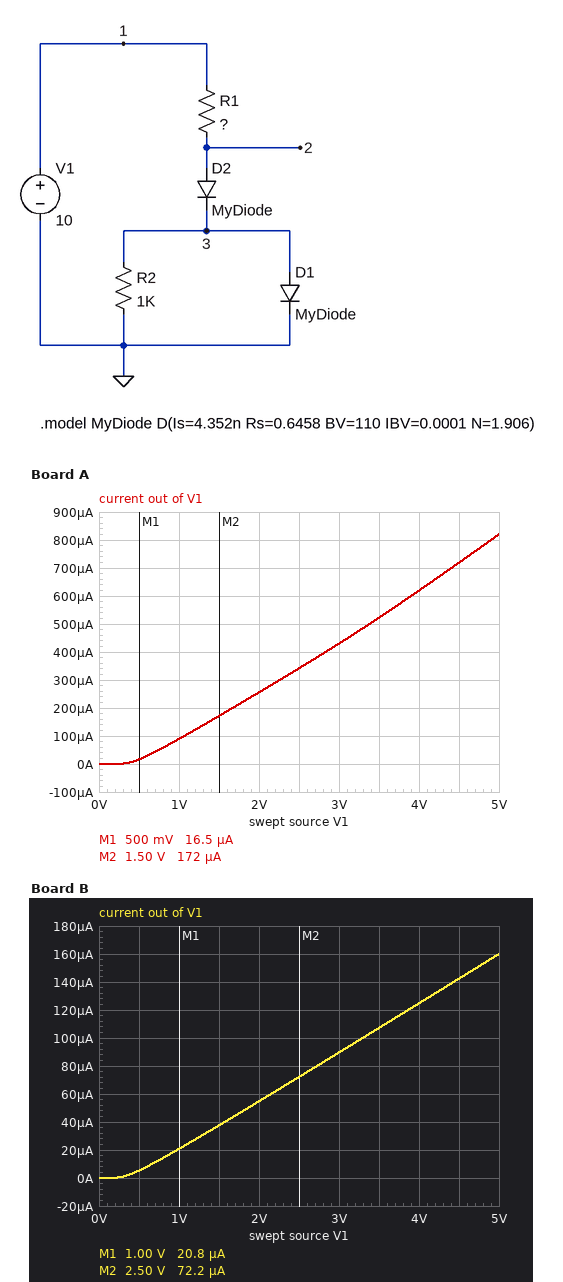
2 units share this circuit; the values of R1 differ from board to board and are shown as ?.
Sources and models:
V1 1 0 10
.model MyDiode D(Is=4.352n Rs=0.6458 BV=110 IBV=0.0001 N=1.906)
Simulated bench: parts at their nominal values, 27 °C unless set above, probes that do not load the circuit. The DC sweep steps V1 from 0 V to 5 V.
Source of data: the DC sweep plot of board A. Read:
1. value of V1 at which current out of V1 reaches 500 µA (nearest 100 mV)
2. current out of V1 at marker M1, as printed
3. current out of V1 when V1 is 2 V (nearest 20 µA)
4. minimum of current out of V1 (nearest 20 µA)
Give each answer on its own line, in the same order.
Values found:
3.4 V
16.5 µA
260 µA
0 A
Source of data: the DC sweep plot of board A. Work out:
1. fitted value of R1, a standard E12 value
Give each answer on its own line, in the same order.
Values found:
4.7 kΩ
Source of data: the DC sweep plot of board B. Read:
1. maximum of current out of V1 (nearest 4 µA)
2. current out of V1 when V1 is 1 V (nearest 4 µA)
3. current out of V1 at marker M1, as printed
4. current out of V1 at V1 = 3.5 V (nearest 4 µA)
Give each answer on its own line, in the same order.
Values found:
160 µA
20 µA
20.8 µA
108 µA
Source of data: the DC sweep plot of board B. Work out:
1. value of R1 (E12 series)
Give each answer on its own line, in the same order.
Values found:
27 kΩ
